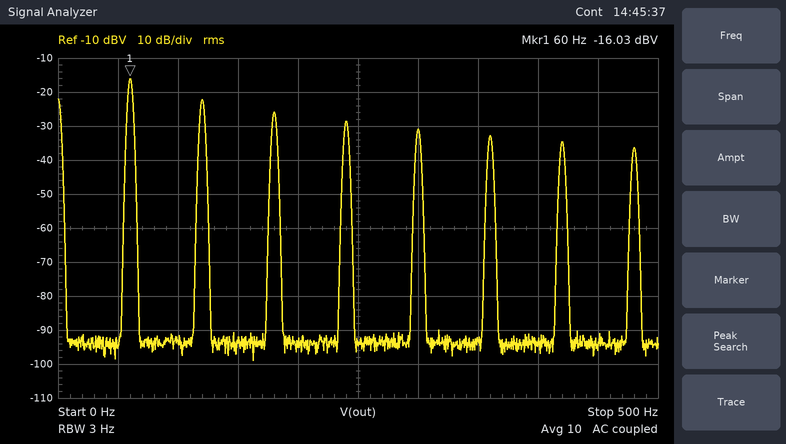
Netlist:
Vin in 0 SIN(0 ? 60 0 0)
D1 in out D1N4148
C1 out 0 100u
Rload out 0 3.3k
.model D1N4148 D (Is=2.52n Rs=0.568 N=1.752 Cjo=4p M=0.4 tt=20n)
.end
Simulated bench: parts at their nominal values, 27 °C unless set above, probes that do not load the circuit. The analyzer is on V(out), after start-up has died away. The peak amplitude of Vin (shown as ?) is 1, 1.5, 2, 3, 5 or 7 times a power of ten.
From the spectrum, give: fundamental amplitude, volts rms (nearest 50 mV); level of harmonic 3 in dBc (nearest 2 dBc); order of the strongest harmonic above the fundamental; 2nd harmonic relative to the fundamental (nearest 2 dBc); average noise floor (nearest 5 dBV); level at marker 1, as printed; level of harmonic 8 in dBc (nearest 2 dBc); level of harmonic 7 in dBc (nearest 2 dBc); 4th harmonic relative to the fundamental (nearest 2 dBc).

150 mV
-10 dBc
2
-6 dBc
-95 dBV
-16.03 dBV
-20 dBc
-18 dBc
-12 dBc
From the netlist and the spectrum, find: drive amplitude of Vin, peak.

15 V
